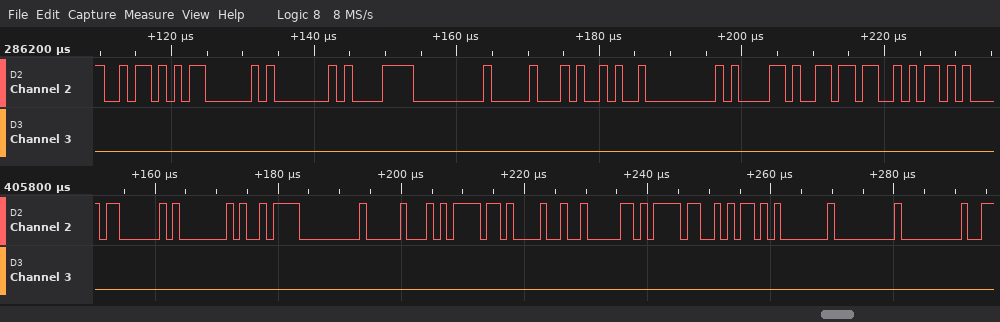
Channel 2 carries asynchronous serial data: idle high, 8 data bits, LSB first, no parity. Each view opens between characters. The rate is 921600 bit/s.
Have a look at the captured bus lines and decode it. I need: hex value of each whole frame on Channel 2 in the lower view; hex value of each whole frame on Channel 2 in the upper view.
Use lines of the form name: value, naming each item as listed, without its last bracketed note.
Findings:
hex value of each whole frame on Channel 2 in the lower view: 03, 01, E9, 00, 10, BD, 21, 82, BD, 6A, 01, 00, 00
hex value of each whole frame on Channel 2 in the upper view: 5A, 03, 01, E1, 00, 10, 29, 00, 61, B6, 6A
